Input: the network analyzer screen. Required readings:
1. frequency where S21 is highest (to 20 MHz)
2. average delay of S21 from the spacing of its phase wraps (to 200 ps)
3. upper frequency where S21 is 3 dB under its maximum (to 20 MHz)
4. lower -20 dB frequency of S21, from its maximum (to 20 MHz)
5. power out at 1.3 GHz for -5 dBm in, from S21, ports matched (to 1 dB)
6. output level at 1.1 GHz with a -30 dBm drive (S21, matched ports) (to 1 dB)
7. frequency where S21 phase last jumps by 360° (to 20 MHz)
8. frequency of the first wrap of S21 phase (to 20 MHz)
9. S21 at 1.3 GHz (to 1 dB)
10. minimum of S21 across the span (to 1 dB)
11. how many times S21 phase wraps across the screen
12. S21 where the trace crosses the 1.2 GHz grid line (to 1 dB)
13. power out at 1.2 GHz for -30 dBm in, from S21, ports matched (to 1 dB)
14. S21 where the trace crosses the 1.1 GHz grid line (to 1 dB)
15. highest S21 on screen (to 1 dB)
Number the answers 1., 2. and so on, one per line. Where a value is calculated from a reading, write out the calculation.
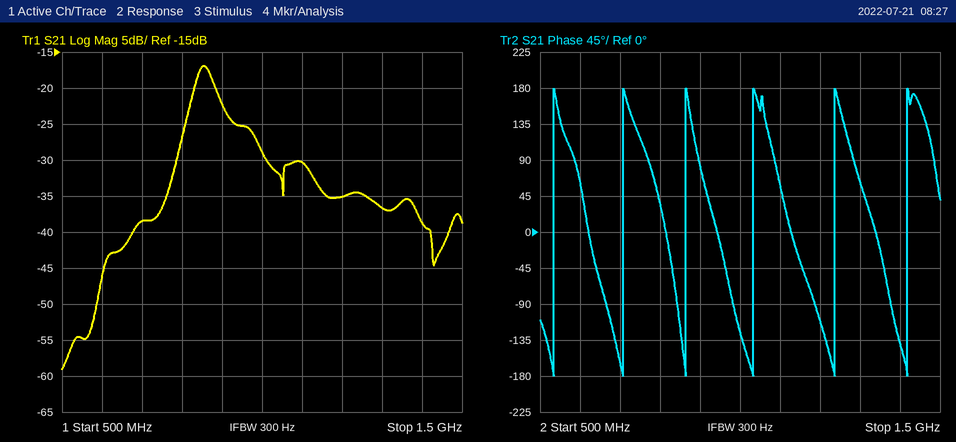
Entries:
1. 860 MHz
2. 5 cycles / (1.42 GHz − 540 MHz) ≈ 5.68 ns, so 5.6 ns to the nearest 200 ps
3. 880 MHz
4. 740 MHz
5. -5 dBm + (-37 dB) = -42 dBm
6. -30 dBm + (-30 dB) = -60 dBm
7. 1.42 GHz
8. 540 MHz
9. -37 dB
10. -59 dB
11. 6
12. -35 dB
13. -30 dBm + (-35 dB) = -65 dBm
14. -30 dB
15. -17 dB
